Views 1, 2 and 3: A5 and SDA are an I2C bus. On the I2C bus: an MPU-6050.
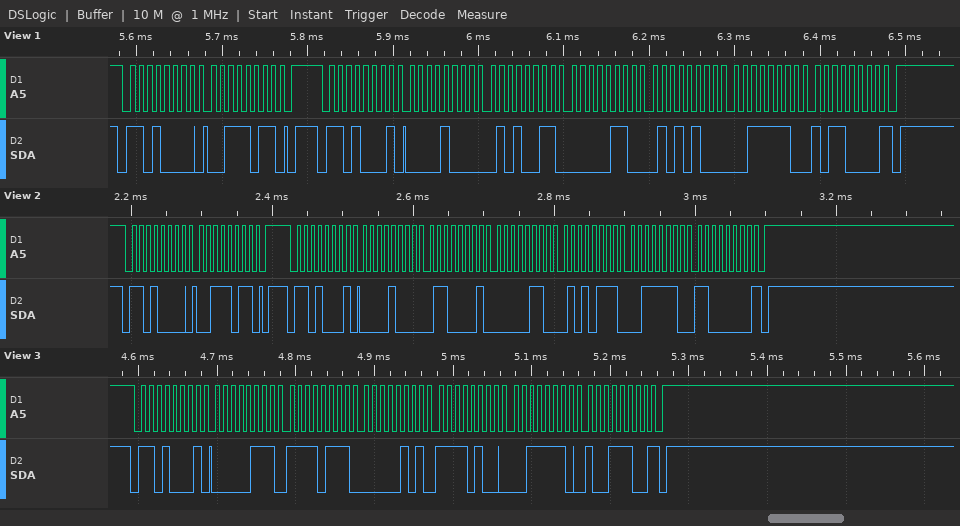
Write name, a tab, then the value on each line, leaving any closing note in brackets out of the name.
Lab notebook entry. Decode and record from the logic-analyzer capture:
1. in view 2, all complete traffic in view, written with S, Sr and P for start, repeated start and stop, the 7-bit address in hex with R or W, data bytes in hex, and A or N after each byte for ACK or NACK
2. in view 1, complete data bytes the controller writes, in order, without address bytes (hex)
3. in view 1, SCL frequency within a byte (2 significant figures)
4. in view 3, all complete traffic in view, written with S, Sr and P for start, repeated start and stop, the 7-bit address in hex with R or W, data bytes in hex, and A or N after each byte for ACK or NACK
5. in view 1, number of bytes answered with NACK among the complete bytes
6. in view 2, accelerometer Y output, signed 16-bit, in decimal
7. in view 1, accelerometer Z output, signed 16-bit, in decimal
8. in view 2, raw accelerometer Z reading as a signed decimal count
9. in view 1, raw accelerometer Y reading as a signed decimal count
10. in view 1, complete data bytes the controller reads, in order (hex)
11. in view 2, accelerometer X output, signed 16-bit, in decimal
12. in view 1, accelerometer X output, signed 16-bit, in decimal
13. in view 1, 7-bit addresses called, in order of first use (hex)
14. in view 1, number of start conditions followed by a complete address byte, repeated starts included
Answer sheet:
in view 2, all complete traffic in view, written with S, Sr and P for start, repeated start and stop, the 7-bit address in hex with R or W, data bytes in hex, and A or N after each byte for ACK or NACK	S 68W A 3B A P S 68R A 08 A 61 A 06 A 57 A 3E A C0 N P
in view 1, complete data bytes the controller writes, in order, without address bytes	3B
in view 1, SCL frequency within a byte	100 kHz
in view 3, all complete traffic in view, written with S, Sr and P for start, repeated start and stop, the 7-bit address in hex with R or W, data bytes in hex, and A or N after each byte for ACK or NACK	S 68R A 07 A F7 A 05 A F4 A 3E A 9C N P
in view 1, number of bytes answered with NACK among the complete bytes	1
in view 2, accelerometer Y output, signed 16-bit, in decimal	1623
in view 1, accelerometer Z output, signed 16-bit, in decimal	16048
in view 2, raw accelerometer Z reading as a signed decimal count	16064
in view 1, raw accelerometer Y reading as a signed decimal count	1620
in view 1, complete data bytes the controller reads, in order	08 53 06 54 3E B0
in view 2, accelerometer X output, signed 16-bit, in decimal	2145
in view 1, accelerometer X output, signed 16-bit, in decimal	2131
in view 1, 7-bit addresses called, in order of first use	0x68
in view 1, number of start conditions followed by a complete address byte, repeated starts included	2
